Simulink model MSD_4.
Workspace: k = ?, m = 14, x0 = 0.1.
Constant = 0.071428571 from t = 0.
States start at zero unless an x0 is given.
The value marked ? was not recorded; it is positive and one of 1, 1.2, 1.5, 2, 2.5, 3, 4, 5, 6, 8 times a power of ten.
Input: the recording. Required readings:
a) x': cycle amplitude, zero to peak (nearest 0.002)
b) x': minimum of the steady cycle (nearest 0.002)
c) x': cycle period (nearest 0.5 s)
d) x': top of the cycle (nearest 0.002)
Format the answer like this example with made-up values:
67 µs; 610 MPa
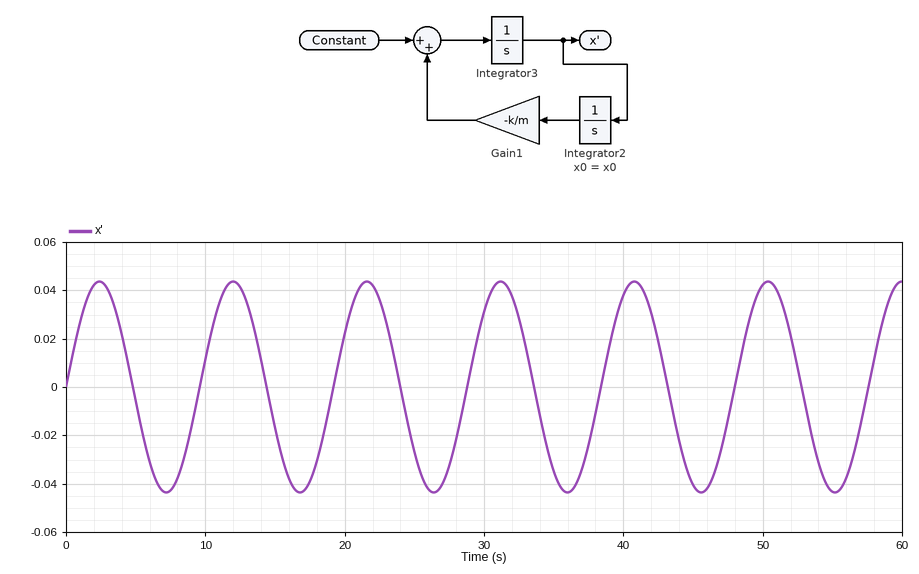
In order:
0.044; -0.044; 9.5 s; 0.044
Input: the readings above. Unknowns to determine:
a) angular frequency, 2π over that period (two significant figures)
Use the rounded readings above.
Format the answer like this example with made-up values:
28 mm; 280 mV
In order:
0.66 rad/s
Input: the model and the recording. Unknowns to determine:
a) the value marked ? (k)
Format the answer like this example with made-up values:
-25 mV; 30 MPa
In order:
6
